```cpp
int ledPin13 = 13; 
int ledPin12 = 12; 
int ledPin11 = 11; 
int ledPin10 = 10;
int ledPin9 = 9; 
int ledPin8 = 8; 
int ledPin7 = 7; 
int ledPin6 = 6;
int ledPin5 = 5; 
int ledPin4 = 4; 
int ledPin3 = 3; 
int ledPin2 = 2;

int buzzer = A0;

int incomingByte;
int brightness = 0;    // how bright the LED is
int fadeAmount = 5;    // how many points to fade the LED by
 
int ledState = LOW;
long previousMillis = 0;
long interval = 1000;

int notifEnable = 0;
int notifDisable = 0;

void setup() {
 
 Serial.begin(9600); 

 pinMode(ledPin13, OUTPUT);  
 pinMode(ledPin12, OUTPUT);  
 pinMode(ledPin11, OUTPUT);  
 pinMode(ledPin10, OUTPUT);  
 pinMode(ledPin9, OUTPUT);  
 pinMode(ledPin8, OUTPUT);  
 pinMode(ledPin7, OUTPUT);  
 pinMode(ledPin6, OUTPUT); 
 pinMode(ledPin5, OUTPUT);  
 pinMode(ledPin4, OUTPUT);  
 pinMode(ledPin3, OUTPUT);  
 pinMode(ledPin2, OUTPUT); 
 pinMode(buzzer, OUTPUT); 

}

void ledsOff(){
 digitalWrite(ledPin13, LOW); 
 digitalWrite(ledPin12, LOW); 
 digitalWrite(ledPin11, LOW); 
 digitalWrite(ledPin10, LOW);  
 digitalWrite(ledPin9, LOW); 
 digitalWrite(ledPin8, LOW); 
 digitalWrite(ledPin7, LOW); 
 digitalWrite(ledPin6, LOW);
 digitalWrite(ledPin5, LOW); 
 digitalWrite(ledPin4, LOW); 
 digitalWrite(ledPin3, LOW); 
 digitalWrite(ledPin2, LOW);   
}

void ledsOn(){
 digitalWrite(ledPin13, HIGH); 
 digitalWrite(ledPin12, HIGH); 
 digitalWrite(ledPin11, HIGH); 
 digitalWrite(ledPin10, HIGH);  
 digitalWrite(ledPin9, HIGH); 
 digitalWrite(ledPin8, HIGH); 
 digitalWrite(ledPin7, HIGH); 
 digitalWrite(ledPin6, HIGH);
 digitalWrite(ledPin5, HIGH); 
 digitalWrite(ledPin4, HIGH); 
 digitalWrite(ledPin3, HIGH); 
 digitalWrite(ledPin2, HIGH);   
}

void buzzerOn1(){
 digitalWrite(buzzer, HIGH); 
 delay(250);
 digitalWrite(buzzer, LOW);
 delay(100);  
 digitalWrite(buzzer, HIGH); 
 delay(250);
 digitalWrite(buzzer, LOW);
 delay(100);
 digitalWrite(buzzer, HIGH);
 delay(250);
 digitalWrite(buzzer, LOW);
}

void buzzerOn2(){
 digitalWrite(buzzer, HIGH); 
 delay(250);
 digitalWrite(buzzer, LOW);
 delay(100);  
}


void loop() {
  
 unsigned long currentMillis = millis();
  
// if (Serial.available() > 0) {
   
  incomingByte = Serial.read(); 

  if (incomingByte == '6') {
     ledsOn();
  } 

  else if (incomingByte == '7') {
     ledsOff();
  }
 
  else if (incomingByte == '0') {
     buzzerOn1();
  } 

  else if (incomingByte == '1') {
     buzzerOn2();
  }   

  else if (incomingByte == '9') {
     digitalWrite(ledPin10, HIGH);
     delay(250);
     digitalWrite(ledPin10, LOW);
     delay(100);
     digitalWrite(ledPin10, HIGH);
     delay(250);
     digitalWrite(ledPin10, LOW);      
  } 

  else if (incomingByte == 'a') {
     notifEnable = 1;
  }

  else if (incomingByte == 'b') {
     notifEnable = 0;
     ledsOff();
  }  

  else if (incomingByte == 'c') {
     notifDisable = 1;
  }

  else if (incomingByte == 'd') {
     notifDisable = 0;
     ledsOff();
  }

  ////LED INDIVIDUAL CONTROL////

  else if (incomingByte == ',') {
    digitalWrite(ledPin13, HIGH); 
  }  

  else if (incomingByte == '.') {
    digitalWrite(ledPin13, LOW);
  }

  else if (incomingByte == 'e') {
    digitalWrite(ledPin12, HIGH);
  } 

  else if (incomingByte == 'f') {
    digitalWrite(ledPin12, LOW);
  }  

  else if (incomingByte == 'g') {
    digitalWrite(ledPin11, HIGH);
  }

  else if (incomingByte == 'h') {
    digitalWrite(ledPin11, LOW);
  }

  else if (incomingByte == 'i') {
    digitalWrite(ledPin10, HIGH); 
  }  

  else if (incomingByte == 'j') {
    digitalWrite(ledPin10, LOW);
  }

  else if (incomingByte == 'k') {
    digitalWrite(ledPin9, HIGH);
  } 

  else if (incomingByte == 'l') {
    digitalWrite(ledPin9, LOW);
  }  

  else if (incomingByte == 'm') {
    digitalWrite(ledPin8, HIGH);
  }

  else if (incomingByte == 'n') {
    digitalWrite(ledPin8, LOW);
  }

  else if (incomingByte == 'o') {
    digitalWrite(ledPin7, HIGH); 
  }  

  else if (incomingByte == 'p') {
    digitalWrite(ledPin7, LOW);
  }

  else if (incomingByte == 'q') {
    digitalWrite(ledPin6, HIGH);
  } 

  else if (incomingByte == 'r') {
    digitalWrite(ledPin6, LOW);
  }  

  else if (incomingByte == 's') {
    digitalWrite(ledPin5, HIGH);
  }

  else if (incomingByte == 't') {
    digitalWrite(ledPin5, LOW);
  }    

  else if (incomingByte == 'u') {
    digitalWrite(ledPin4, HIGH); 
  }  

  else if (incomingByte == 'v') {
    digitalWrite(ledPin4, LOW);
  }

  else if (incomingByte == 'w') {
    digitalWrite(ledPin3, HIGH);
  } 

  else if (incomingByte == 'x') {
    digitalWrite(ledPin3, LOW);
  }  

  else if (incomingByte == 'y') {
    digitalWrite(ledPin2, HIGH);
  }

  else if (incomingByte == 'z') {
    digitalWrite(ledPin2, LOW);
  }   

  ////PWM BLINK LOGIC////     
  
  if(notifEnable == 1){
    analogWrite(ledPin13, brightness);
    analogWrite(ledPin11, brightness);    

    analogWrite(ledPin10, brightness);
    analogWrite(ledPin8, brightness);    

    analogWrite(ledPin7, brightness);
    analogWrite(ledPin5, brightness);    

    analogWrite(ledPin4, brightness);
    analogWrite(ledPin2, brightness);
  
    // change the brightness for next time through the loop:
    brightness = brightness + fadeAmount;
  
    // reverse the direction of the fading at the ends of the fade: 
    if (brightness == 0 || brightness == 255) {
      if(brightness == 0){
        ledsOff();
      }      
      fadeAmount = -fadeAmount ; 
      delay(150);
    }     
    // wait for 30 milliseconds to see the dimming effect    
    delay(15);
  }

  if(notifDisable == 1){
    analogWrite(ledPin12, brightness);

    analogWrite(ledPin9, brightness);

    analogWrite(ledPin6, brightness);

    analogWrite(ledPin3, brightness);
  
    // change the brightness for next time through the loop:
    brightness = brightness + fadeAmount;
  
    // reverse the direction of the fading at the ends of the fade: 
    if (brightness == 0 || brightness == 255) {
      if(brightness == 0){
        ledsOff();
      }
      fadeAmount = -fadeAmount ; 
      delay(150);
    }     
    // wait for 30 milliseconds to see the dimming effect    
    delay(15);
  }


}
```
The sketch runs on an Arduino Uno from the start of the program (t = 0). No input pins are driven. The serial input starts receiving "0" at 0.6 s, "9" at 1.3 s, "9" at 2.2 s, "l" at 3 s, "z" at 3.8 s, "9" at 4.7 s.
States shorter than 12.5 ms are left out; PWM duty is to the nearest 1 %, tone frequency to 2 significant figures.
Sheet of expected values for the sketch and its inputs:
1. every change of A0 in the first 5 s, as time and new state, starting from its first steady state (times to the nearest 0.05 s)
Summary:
0 s low; 0.6 s high; 0.85 s low; 0.95 s high; 1.2 s low; 1.3 s high; 1.55 s low
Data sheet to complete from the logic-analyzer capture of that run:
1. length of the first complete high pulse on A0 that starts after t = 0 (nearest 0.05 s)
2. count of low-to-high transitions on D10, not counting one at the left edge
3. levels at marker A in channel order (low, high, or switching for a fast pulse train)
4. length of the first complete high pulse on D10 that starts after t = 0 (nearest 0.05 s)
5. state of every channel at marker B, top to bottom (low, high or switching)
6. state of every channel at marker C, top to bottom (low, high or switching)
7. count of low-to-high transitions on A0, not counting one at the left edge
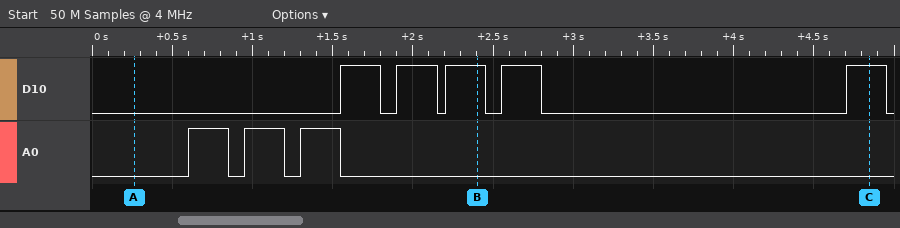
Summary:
0.25 s
5
D10 low, A0 low
0.25 s
D10 high, A0 low
D10 high, A0 low
3
